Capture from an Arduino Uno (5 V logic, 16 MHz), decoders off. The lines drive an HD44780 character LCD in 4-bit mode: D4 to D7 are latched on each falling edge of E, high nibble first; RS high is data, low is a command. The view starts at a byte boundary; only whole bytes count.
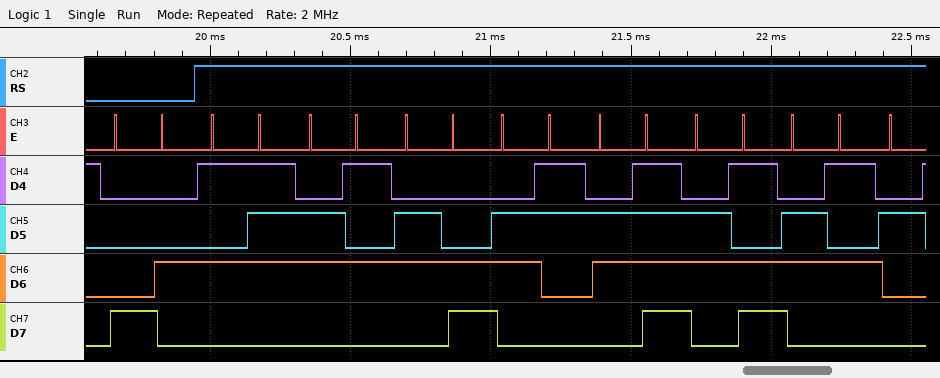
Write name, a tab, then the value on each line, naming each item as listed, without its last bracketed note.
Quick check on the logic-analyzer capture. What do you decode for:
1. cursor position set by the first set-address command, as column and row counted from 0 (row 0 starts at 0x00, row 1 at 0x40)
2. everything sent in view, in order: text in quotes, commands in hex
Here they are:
cursor position set by the first set-address command, as column and row counted from 0	column 4, row 0
everything sent in view, in order: text in quotes, commands in hex	0x84 "Welcome"
